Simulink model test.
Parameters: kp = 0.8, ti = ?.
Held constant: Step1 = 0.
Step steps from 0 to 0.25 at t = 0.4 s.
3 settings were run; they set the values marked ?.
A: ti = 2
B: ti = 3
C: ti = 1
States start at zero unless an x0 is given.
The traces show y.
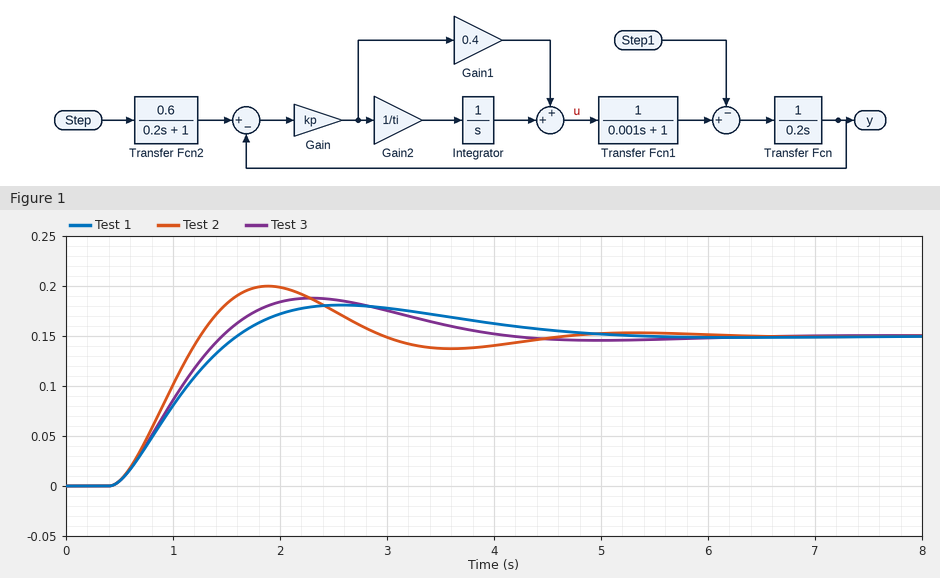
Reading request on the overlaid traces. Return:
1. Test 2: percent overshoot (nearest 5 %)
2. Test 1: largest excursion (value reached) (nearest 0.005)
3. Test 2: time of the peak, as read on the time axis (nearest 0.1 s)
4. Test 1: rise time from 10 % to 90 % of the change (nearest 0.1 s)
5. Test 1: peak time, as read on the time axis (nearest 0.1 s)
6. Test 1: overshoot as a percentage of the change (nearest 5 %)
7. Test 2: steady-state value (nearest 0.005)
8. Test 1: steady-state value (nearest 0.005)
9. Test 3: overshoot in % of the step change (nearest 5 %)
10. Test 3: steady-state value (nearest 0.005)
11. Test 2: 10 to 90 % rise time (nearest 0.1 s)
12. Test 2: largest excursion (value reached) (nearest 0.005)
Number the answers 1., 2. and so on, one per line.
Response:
1. 35 %
2. 0.180
3. 1.9 s
4. 0.8 s
5. 2.6 s
6. 20 %
7. 0.150
8. 0.150
9. 25 %
10. 0.150
11. 0.6 s
12. 0.200
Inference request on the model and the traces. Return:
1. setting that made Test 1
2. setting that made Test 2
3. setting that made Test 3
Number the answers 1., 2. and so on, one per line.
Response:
1. B
2. C
3. A
